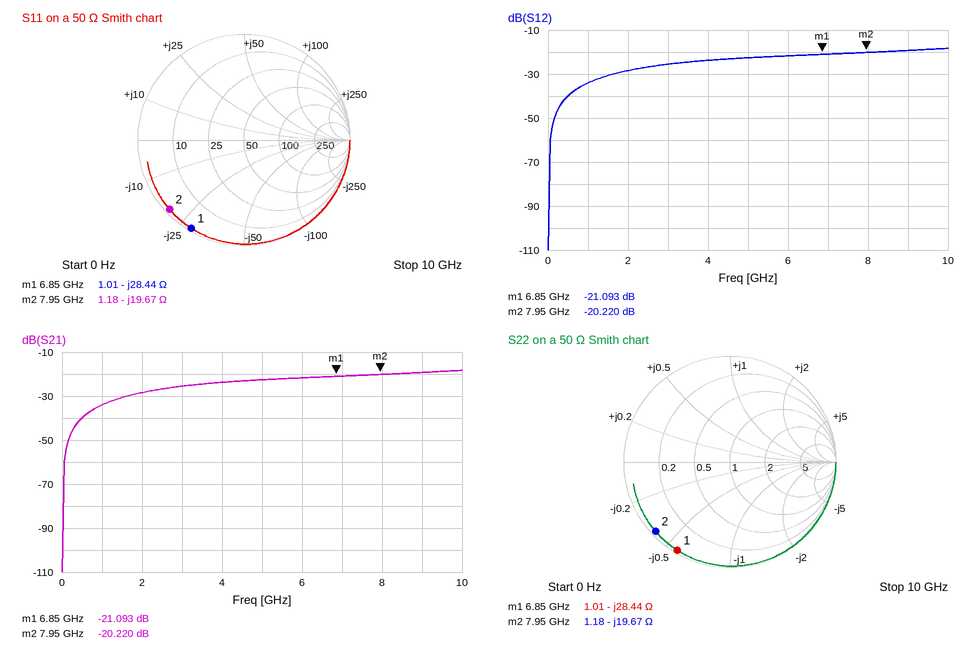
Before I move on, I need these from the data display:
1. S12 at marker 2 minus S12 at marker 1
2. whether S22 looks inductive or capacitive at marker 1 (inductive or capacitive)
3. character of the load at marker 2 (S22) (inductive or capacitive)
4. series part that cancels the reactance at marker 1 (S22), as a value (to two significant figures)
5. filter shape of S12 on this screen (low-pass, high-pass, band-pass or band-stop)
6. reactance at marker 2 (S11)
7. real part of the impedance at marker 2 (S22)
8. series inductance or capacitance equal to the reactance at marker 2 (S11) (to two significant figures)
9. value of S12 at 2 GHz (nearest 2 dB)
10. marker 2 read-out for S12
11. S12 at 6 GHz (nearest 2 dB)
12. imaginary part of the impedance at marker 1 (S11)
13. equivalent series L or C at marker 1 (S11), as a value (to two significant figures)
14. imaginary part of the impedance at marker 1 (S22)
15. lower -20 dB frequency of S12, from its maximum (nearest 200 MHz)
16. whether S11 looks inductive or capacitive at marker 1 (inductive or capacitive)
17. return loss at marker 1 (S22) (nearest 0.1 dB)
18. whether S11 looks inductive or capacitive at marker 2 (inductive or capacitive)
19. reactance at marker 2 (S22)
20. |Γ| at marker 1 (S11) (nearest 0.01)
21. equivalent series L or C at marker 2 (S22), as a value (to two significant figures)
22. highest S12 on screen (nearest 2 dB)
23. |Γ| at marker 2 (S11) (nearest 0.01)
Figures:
0.873 dB
capacitive
capacitive
660 pH
high-pass
-19.67 Ω
1.18 Ω
1.0 pF
-28 dB
-20.220 dB
-22 dB
-28.44 Ω
820 fF
-28.44 Ω
600 MHz
capacitive
0.3 dB
capacitive
-19.67 Ω
0.97
1.0 pF
-18 dB
0.96
